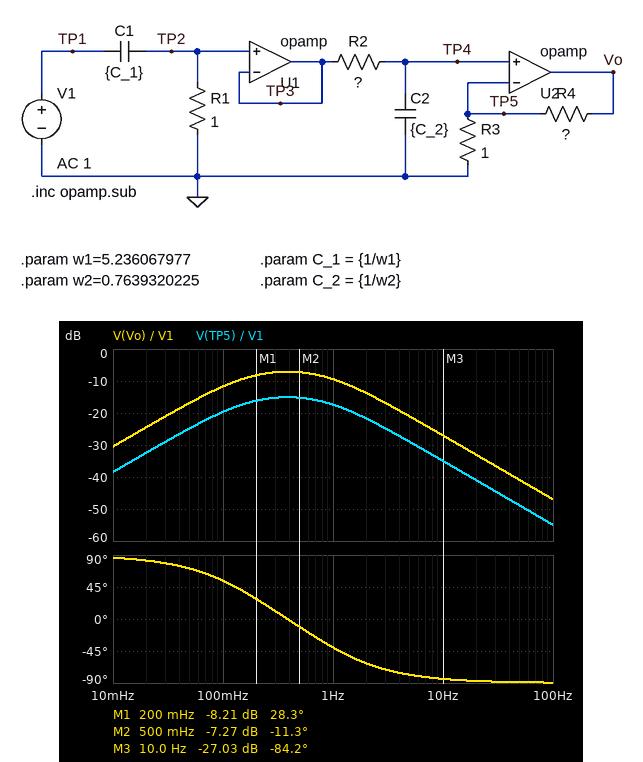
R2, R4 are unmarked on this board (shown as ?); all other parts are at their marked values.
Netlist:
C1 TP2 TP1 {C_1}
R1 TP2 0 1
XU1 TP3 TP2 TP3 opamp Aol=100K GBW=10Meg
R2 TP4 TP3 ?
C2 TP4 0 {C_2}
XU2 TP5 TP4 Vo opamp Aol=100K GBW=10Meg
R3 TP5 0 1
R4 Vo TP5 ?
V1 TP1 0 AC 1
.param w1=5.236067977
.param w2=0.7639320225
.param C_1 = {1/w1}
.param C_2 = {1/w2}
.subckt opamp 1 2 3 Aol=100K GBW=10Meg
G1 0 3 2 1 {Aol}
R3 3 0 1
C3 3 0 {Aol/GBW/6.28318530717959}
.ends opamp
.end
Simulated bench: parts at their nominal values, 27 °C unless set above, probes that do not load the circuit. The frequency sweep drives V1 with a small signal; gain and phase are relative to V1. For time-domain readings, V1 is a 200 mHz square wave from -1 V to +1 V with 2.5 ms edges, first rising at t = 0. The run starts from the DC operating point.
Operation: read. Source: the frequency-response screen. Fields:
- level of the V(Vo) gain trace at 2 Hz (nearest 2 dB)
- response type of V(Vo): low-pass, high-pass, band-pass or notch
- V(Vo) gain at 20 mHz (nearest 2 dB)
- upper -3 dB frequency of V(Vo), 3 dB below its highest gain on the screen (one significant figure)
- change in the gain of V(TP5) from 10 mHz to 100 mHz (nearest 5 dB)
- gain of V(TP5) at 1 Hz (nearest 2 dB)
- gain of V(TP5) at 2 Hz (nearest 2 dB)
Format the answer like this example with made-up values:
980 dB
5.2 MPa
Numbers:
-14 dB
band-pass
-24 dB
1 Hz
20 dB
-18 dB
-22 dB
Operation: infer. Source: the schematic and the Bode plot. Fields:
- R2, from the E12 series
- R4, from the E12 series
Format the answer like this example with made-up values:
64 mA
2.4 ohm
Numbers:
0.68 Ω
1.5 Ω
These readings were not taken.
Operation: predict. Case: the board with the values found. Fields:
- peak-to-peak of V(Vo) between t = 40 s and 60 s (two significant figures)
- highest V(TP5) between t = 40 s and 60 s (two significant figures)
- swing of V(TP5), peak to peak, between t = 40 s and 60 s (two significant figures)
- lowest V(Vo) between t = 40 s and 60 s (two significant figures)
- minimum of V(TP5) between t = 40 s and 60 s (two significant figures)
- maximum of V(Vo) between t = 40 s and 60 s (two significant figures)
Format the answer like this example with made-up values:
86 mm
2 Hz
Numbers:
1.3 V
260 mV
520 mV
-650 mV
-260 mV
650 mV
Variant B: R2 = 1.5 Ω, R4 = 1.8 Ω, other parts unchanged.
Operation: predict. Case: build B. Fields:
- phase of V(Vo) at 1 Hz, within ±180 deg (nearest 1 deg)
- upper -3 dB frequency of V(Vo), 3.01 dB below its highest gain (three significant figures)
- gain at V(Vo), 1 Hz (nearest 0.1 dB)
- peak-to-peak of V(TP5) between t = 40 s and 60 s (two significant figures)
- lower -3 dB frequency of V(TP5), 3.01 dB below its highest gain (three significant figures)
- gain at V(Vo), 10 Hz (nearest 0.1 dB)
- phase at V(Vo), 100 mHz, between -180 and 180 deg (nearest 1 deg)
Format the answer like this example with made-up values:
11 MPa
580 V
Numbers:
-46 deg
983 mHz
-15.2 dB
230 mV
68.7 mHz
-32.9 dB
32 deg
